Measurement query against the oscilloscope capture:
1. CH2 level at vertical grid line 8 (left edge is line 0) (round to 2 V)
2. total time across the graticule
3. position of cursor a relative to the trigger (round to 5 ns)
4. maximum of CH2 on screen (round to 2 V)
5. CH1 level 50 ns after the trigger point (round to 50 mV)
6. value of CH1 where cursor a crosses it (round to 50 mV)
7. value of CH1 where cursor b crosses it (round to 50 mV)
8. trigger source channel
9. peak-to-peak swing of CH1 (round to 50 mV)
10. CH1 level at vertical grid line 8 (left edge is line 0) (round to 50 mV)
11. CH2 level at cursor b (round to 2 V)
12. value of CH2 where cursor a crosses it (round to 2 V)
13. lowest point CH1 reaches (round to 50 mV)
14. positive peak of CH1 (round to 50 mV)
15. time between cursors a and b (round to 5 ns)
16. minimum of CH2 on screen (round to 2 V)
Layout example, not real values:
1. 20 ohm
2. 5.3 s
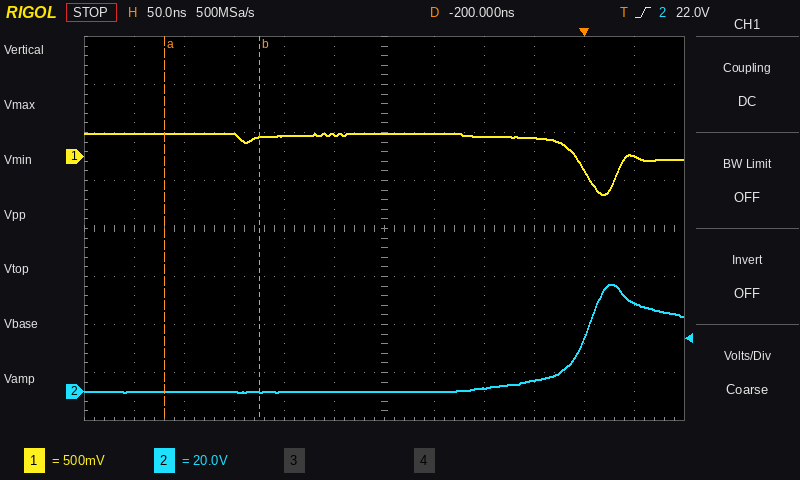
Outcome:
1. 2 V
2. 600 ns
3. -420 ns
4. 44 V
5. 0 mV
6. 250 mV
7. 200 mV
8. CH2
9. 650 mV
10. 200 mV
11. 0 V
12. 0 V
13. -400 mV
14. 250 mV
15. 95 ns
16. 0 V
